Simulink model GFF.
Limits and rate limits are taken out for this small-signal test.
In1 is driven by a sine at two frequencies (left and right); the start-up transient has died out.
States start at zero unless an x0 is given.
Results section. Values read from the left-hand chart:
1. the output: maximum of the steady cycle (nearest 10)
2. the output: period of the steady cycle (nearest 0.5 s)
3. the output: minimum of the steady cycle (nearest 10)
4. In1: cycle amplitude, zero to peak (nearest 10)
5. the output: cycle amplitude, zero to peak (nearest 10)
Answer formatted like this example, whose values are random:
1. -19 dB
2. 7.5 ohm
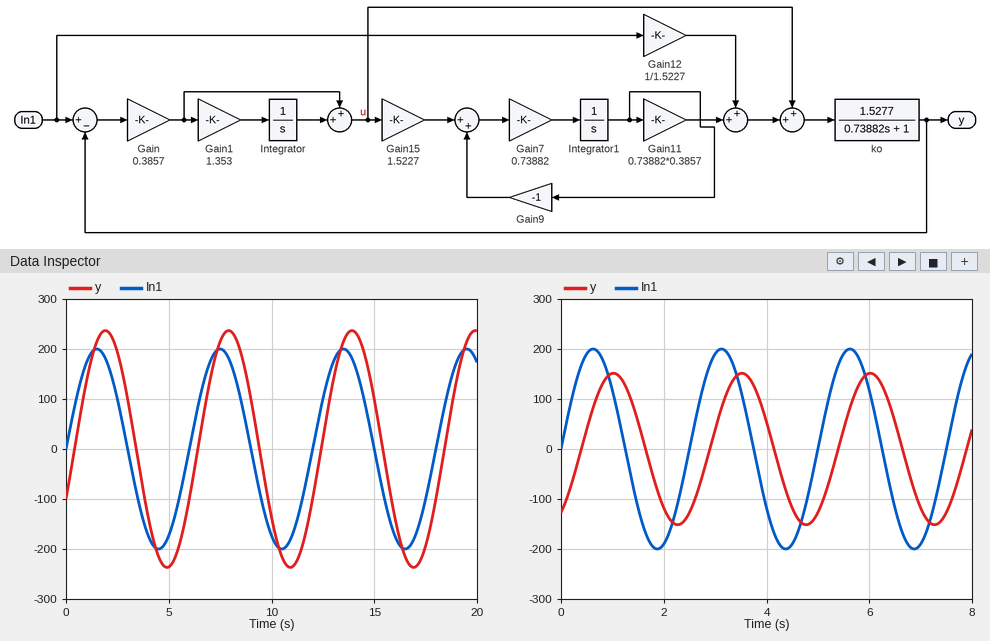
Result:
1. 240
2. 6.0 s
3. -240
4. 200
5. 240
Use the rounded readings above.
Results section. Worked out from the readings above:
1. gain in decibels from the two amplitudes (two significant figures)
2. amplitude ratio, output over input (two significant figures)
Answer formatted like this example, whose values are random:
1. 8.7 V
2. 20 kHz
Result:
1. 1.6 dB
2. 1.2
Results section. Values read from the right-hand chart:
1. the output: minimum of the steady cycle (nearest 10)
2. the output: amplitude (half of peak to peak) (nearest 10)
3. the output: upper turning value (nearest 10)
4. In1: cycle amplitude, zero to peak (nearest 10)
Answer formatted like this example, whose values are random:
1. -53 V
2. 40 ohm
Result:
1. -150
2. 150
3. 150
4. 200
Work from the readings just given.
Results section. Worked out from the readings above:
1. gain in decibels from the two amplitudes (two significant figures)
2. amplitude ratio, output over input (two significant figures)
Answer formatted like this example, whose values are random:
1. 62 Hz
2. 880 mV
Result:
1. -2.5 dB
2. 0.75
